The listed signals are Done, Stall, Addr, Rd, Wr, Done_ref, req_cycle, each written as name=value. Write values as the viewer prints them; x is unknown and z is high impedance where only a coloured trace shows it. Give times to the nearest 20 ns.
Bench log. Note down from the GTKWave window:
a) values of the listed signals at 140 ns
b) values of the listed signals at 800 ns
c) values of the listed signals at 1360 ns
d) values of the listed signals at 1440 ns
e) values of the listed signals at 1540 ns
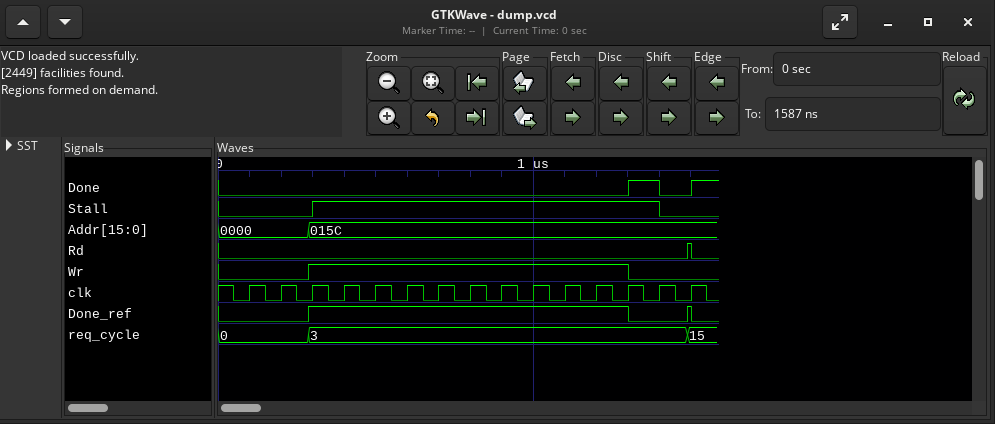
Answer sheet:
Done=0, Stall=0, Addr=0000, Rd=0, Wr=0, Done_ref=0, req_cycle=0
Done=0, Stall=1, Addr=015C, Rd=0, Wr=1, Done_ref=1, req_cycle=3
Done=1, Stall=1, Addr=015C, Rd=0, Wr=0, Done_ref=0, req_cycle=3
Done=0, Stall=0, Addr=015C, Rd=0, Wr=0, Done_ref=0, req_cycle=3
Done=1, Stall=0, Addr=015C, Rd=0, Wr=0, Done_ref=0, req_cycle=15
